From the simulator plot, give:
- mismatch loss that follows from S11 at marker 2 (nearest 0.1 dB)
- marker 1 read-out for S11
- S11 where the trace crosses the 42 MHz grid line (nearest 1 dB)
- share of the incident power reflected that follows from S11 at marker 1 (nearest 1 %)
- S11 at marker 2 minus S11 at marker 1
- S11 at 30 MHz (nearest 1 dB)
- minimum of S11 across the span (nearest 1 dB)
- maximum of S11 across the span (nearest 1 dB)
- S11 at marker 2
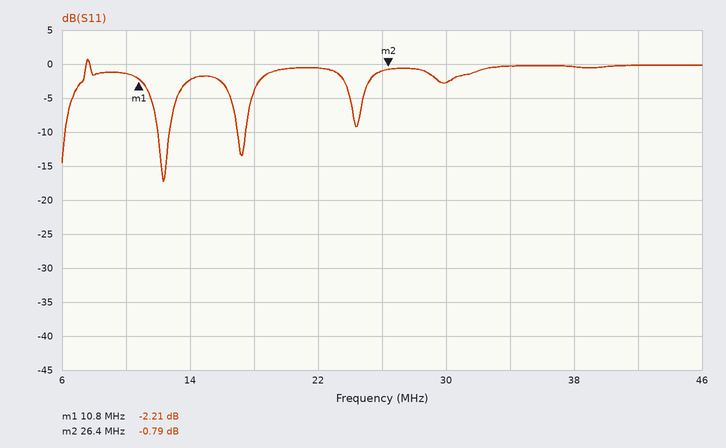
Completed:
7.8 dB
-2.21 dB
0 dB
60 %
1.42 dB
-3 dB
-17 dB
1 dB
-0.79 dB
